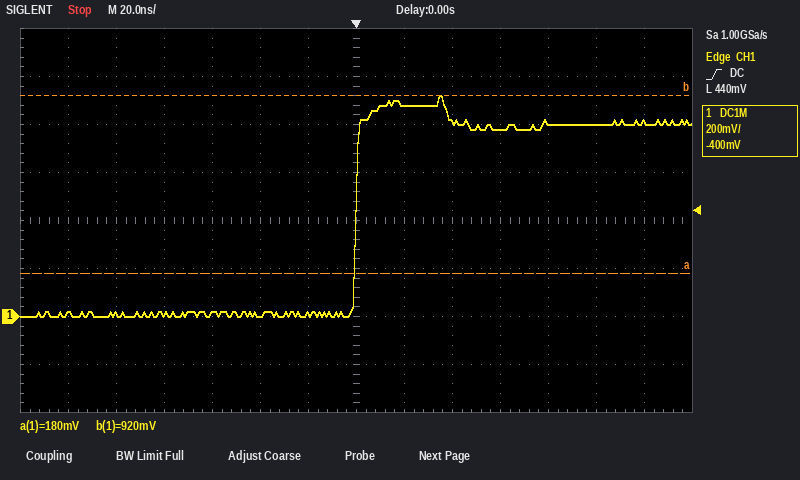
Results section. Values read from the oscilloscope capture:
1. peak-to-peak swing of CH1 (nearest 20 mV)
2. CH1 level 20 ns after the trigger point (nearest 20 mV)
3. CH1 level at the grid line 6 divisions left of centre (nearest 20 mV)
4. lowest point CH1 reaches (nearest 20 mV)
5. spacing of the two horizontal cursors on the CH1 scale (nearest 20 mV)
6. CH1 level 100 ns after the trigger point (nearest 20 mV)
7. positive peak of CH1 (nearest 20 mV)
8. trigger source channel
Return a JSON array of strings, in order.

["920 mV", "880 mV", "20 mV", "0 mV", "740 mV", "800 mV", "920 mV", "CH1"]
